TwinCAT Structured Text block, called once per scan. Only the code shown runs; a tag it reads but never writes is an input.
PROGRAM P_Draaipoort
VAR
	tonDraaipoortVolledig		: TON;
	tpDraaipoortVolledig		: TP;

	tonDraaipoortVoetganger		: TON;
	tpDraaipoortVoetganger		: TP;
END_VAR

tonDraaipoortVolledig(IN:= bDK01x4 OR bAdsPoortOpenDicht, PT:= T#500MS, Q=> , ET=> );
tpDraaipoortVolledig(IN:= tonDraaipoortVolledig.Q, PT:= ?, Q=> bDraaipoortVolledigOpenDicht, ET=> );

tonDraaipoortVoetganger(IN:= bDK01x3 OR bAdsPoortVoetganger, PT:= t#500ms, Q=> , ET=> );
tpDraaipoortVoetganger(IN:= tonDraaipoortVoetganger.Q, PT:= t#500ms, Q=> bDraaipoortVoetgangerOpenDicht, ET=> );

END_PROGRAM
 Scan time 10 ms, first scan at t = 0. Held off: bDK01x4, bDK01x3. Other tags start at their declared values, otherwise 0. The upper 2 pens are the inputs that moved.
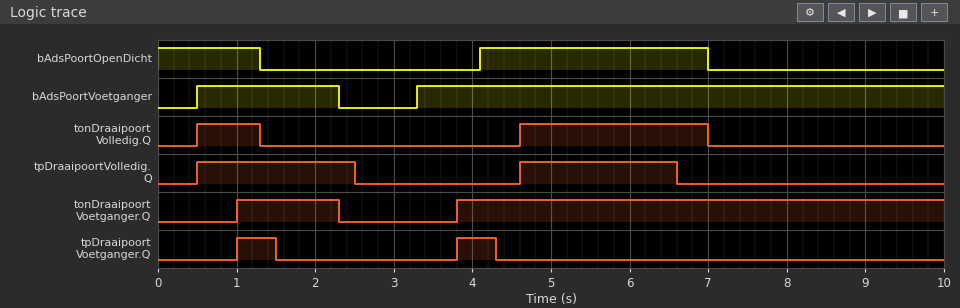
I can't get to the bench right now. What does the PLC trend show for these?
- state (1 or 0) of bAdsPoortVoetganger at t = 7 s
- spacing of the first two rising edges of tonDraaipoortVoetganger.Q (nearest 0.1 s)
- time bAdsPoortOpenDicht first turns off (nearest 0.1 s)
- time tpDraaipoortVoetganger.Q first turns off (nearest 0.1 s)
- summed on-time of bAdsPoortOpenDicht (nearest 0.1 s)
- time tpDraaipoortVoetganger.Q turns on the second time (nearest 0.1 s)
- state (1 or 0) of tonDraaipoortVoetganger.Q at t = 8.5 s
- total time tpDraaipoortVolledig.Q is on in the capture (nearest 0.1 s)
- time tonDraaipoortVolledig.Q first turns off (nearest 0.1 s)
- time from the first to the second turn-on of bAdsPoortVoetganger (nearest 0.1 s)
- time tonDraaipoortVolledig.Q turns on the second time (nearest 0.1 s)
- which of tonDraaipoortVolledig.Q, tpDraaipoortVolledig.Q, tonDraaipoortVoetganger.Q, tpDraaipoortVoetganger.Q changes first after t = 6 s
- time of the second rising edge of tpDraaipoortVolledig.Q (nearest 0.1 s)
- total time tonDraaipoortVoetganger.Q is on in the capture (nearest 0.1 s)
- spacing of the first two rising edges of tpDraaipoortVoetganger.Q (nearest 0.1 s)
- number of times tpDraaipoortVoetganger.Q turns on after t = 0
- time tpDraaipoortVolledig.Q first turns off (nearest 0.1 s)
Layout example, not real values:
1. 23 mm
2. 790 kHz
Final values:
1. 1
2. 2.8 s
3. 1.3 s
4. 1.5 s
5. 4.2 s
6. 3.8 s
7. 1
8. 4.0 s
9. 1.3 s
10. 2.8 s
11. 4.6 s
12. tpDraaipoortVolledig.Q
13. 4.6 s
14. 7.5 s
15. 2.8 s
16. 2
17. 2.5 s
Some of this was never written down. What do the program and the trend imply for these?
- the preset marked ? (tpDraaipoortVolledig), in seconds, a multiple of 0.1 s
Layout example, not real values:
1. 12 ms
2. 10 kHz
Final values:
1. 2.0 s
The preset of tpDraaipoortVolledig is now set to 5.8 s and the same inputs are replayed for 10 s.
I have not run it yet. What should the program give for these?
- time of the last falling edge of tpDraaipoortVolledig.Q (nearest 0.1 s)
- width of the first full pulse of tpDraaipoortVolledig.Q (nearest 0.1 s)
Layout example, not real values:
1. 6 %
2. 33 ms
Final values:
1. 6.3 s
2. 5.8 s
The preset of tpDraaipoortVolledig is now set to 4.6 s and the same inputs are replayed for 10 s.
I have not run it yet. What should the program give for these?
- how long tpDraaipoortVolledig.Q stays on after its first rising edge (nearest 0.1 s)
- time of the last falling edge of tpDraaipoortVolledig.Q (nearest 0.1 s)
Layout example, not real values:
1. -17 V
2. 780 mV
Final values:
1. 4.6 s
2. 5.1 s
